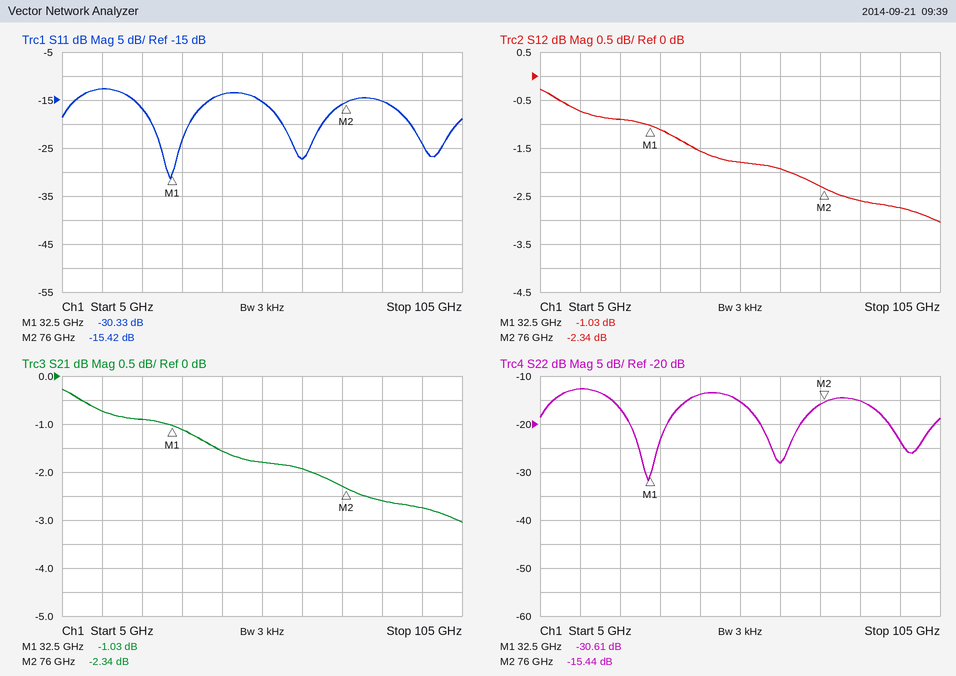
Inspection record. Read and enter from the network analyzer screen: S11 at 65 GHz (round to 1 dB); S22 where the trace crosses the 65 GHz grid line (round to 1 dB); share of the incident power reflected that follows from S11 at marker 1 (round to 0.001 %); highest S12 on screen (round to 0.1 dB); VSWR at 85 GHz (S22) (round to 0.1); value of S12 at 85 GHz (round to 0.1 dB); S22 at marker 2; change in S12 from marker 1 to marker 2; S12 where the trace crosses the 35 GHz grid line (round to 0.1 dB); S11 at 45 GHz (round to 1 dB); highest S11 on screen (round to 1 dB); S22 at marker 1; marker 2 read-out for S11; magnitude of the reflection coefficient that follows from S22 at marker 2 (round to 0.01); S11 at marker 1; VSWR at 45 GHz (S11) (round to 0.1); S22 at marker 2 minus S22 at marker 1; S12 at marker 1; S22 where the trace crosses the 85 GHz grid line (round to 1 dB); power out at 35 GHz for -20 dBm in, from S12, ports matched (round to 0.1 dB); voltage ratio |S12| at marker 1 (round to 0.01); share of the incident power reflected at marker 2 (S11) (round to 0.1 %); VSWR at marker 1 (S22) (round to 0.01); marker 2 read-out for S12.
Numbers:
-27 dB
-28 dB
0.093 %
-0.3 dB
1.4
-2.6 dB
-15.44 dB
-1.31 dB
-1.1 dB
-14 dB
-13 dB
-30.61 dB
-15.42 dB
0.17
-30.33 dB
1.5
15.17 dB
-1.03 dB
-15 dB
-21.1 dBm
0.89
2.9 %
1.06
-2.34 dB
